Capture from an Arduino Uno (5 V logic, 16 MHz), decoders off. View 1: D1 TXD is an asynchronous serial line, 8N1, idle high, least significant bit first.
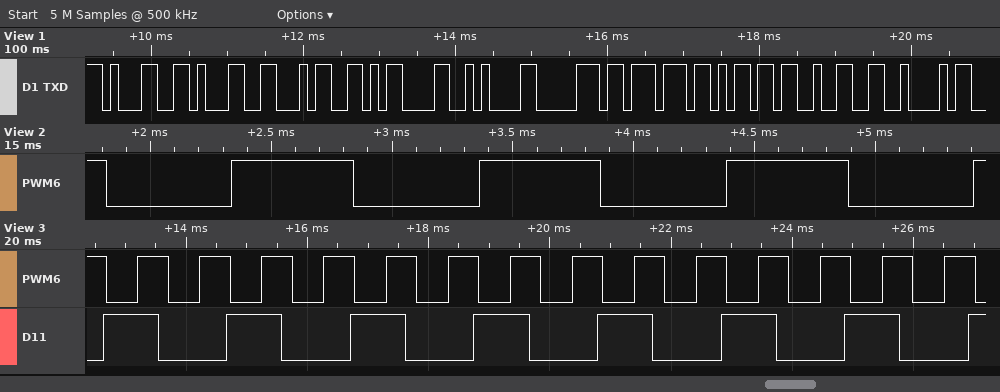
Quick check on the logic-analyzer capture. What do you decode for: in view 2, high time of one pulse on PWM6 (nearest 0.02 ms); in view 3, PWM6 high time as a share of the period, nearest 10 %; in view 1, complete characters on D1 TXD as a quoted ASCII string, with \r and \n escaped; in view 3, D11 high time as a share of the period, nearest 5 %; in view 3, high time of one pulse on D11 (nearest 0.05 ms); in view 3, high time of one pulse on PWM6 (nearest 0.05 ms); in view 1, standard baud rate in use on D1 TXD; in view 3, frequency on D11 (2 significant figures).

0.50 ms
50 %
"114\r\npwm2B"
45 %
0.90 ms
0.50 ms
9600 baud
490 Hz
